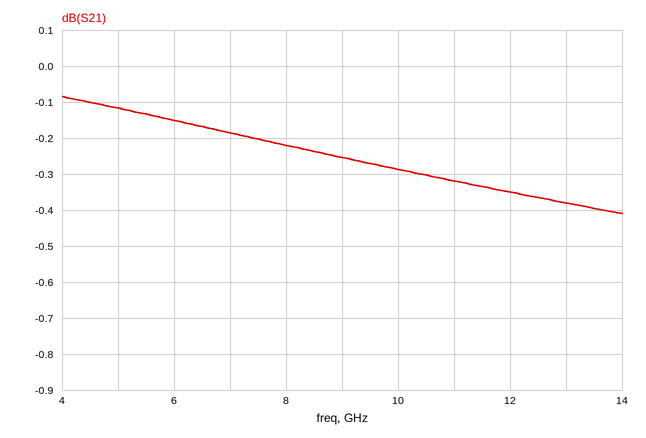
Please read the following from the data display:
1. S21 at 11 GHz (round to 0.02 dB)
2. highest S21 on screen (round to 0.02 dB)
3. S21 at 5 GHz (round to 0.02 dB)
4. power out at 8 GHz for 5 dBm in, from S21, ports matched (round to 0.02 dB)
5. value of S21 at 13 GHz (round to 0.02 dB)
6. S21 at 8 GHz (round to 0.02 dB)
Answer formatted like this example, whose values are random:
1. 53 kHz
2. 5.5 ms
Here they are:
1. -0.32 dB
2. -0.08 dB
3. -0.12 dB
4. 4.78 dBm
5. -0.38 dB
6. -0.22 dB
